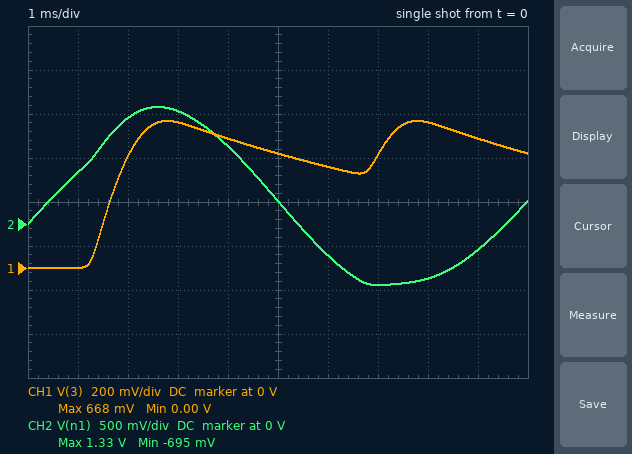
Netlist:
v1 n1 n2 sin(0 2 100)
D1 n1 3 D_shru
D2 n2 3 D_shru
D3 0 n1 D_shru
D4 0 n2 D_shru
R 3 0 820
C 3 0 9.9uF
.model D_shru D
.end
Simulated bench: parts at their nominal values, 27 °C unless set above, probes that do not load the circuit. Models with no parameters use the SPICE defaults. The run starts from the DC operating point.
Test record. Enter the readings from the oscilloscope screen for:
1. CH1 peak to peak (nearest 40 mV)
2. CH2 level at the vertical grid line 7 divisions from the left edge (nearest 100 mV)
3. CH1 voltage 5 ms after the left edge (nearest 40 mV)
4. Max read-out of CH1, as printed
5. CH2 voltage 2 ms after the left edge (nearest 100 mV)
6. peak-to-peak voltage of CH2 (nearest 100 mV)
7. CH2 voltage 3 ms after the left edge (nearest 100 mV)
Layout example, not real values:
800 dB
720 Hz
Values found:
680 mV
-700 mV
520 mV
668 mV
1.2 V
2.0 V
1.3 V
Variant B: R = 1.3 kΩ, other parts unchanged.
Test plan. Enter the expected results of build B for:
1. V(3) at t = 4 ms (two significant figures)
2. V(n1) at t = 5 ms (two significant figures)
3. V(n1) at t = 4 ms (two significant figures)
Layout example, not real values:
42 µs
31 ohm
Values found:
630 mV
290 mV
900 mV
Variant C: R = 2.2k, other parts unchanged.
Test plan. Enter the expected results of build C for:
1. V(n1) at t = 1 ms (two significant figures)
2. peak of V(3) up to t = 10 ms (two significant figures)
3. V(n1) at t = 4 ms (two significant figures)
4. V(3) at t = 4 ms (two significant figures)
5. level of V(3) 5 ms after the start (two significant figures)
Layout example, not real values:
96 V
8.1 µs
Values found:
590 mV
690 mV
920 mV
660 mV
630 mV
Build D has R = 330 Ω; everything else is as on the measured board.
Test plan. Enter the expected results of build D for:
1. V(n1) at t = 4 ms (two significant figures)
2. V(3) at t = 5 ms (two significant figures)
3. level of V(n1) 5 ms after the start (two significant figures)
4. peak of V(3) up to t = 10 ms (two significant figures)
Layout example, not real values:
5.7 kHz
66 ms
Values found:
820 mV
340 mV
170 mV
640 mV
